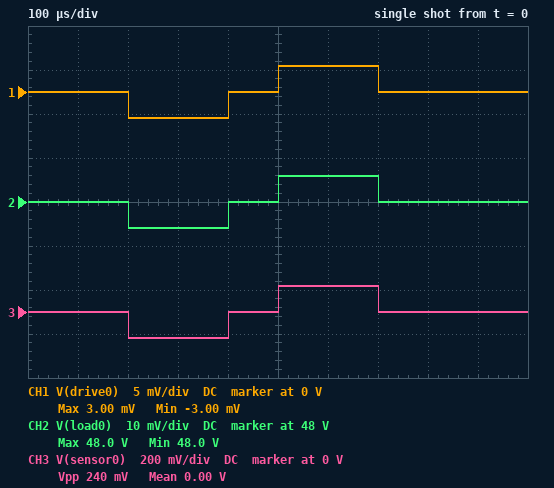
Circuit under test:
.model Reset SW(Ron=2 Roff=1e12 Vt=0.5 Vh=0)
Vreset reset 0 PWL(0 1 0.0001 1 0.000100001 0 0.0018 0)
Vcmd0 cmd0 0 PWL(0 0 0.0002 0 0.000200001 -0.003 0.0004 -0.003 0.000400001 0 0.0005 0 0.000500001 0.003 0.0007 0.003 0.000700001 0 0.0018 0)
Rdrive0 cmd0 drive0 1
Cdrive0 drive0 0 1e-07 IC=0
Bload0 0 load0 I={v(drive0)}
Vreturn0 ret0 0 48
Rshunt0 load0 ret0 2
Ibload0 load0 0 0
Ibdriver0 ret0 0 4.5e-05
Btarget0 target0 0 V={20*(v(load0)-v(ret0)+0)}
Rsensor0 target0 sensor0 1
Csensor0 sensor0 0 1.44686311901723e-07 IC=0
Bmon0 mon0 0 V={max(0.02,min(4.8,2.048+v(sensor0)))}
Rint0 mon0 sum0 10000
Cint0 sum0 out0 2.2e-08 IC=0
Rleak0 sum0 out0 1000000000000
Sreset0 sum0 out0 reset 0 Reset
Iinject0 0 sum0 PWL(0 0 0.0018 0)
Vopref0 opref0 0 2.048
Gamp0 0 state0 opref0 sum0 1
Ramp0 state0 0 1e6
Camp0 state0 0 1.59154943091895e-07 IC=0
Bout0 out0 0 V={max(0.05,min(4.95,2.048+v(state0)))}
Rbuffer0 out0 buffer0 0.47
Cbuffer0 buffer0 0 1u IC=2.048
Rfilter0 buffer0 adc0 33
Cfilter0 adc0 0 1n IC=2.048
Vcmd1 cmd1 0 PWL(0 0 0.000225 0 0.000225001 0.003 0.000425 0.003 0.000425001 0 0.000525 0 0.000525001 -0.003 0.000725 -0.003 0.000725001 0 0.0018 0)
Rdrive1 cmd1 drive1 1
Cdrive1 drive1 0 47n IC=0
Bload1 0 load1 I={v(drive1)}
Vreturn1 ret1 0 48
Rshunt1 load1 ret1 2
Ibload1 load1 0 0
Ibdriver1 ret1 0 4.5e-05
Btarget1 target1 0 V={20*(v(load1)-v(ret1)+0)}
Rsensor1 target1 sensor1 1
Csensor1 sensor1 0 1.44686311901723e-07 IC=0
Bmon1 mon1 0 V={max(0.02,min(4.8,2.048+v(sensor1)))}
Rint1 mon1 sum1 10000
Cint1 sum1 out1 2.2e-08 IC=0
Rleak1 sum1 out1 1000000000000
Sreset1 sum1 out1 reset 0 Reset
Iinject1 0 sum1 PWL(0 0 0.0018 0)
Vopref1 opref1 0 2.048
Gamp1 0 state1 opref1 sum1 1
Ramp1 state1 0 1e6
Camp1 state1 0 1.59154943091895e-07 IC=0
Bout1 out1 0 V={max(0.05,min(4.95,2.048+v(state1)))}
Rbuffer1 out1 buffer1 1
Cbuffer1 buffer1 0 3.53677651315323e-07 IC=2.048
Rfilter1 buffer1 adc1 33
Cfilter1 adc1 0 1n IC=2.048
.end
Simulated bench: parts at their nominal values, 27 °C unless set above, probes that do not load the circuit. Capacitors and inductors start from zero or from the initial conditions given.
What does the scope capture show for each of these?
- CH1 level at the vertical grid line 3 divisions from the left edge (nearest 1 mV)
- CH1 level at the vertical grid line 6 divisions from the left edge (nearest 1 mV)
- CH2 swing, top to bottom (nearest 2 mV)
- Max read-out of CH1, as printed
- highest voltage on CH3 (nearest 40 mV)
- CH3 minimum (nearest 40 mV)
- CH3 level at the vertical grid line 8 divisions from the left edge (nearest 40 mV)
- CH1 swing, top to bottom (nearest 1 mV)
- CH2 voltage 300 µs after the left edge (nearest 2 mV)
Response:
-3 mV
3 mV
12 mV
3.00 mV
120 mV
-120 mV
0 V
6 mV
47.994 V
